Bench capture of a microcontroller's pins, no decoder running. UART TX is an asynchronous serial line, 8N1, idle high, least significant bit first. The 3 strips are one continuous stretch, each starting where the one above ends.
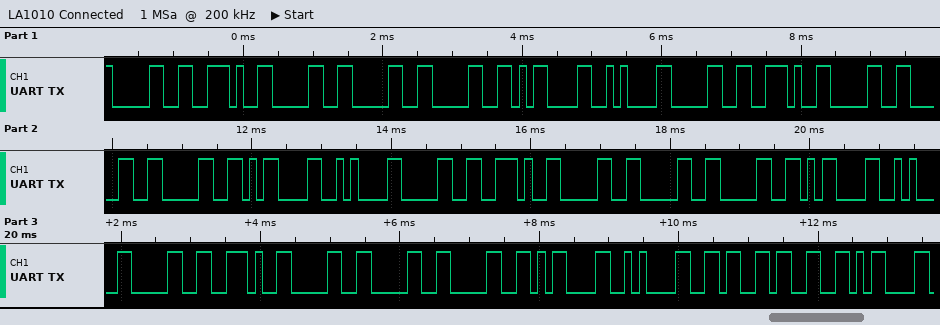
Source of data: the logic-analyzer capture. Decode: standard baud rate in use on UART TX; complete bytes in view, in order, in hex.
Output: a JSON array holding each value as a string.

["9600 baud", "30 2E 30 30 30 0D 0A 30 2E 30 30 30 0D 0A 30 2E 30 30 30 0D 0A 30 2E 30 30 30 0D 0A 36 33 0D"]
